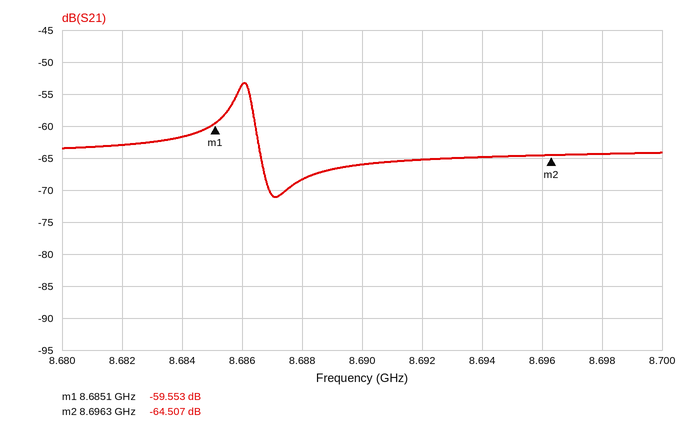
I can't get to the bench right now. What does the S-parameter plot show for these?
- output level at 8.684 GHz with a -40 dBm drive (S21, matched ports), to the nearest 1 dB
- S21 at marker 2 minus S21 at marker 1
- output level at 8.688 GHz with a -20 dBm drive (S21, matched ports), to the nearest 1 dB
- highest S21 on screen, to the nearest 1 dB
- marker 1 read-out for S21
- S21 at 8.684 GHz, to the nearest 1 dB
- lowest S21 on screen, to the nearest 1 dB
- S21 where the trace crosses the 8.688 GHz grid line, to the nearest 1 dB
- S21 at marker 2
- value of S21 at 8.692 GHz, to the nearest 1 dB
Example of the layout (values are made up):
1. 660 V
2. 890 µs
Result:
1. -102 dBm
2. -4.954 dB
3. -88 dBm
4. -53 dB
5. -59.553 dB
6. -62 dB
7. -71 dB
8. -68 dB
9. -64.507 dB
10. -65 dB
